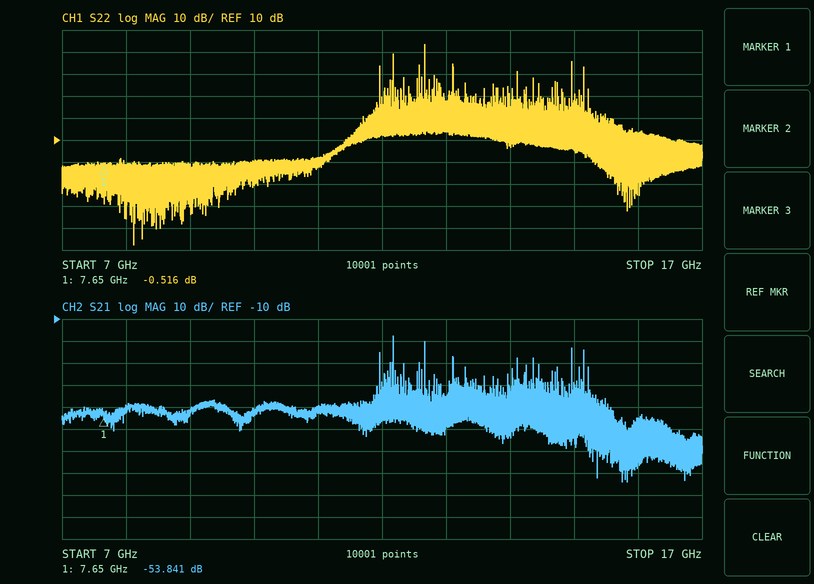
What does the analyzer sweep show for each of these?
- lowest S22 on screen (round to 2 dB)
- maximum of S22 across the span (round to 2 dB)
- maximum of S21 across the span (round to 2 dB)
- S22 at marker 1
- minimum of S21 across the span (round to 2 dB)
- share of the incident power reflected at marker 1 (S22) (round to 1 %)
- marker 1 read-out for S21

-38 dB
54 dB
-18 dB
-0.516 dB
-84 dB
89 %
-53.841 dB
